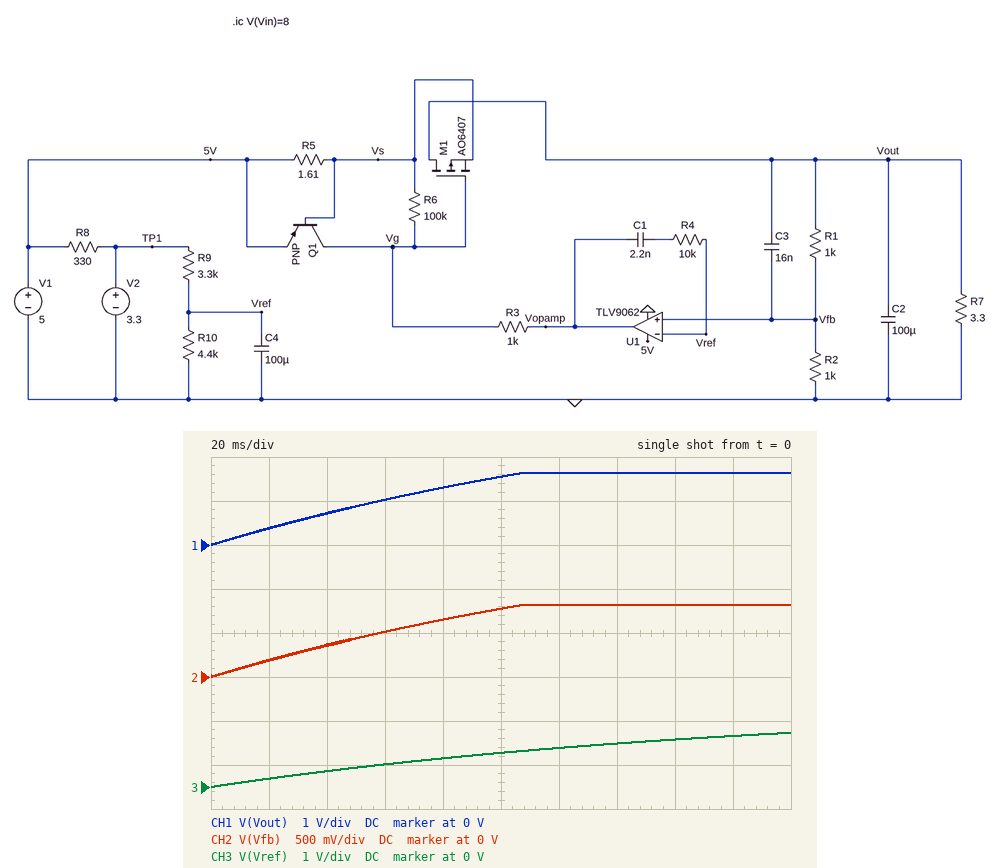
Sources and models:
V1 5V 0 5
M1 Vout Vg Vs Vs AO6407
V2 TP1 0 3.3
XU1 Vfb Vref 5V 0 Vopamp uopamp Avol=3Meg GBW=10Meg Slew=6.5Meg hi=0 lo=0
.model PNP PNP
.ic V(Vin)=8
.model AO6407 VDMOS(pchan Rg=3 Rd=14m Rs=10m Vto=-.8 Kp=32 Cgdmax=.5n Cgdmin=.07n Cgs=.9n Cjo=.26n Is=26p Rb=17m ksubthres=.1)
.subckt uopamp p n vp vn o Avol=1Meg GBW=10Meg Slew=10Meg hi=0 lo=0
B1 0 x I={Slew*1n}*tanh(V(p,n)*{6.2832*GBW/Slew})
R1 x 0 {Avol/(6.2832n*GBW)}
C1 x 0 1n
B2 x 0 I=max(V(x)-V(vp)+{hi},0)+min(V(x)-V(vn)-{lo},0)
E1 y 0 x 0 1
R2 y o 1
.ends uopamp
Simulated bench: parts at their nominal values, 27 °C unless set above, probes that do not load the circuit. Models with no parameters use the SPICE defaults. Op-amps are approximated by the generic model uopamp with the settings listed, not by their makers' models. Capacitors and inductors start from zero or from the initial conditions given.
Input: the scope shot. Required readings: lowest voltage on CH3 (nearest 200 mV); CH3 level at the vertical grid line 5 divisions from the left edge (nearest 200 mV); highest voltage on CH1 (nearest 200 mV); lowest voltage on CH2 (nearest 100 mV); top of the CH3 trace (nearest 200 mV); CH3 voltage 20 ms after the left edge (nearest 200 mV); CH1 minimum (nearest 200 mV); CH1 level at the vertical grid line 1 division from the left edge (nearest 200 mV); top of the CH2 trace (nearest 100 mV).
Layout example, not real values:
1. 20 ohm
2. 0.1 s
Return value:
1. 0 V
2. 800 mV
3. 1.6 V
4. 0 V
5. 1.2 V
6. 200 mV
7. 0 V
8. 400 mV
9. 800 mV
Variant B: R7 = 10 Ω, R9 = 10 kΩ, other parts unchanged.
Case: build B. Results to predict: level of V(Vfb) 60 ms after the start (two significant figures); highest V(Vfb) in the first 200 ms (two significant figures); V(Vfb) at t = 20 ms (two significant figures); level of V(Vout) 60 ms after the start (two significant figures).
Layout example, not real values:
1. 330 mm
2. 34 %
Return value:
1. 180 mV
2. 480 mV
3. 64 mV
4. 360 mV
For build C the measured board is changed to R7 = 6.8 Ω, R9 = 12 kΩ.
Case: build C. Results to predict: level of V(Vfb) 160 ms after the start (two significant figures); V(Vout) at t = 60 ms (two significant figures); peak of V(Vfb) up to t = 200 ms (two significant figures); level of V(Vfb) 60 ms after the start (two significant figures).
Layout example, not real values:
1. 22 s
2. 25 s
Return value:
1. 350 mV
2. 300 mV
3. 410 mV
4. 150 mV
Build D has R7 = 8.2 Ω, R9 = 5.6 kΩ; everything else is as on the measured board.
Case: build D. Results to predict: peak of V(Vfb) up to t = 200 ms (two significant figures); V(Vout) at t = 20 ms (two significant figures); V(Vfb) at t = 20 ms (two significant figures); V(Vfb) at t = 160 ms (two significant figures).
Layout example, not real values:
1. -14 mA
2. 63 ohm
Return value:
1. 810 mV
2. 230 mV
3. 110 mV
4. 690 mV
